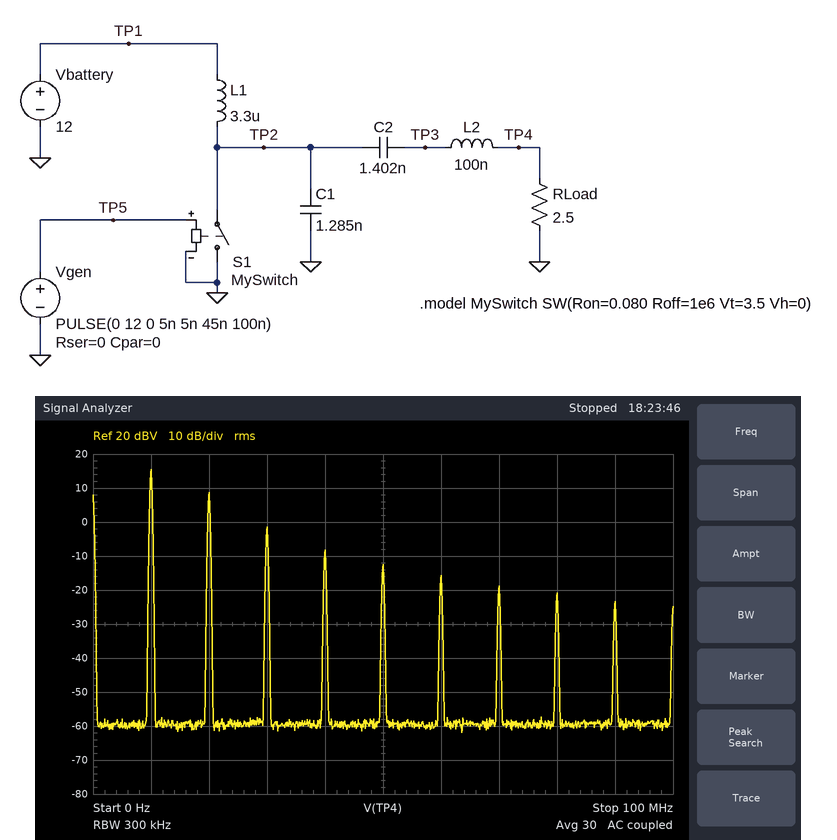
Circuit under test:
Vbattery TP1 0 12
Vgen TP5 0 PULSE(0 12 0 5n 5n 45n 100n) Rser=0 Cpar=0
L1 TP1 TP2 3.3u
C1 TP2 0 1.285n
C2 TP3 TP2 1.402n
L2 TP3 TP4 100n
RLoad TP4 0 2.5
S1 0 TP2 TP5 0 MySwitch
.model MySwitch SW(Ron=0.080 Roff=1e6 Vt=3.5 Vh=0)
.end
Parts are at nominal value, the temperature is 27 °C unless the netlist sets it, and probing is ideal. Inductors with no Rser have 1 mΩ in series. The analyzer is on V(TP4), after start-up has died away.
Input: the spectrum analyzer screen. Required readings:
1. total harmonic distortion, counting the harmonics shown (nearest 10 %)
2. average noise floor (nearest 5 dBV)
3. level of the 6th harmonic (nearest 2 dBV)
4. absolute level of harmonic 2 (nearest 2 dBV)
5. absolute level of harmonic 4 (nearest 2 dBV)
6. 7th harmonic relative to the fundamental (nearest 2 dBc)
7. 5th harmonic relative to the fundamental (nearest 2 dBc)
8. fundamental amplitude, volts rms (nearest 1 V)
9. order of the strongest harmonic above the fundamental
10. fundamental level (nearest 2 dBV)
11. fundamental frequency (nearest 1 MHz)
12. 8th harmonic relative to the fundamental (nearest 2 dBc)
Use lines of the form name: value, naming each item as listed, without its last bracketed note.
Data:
total harmonic distortion, counting the harmonics shown: 50 %
average noise floor: -60 dBV
level of the 6th harmonic: -16 dBV
absolute level of harmonic 2: 8 dBV
absolute level of harmonic 4: -8 dBV
7th harmonic relative to the fundamental: -34 dBc
5th harmonic relative to the fundamental: -28 dBc
fundamental amplitude, volts rms: 6 V
order of the strongest harmonic above the fundamental: 2
fundamental level: 16 dBV
fundamental frequency: 10 MHz
8th harmonic relative to the fundamental: -36 dBc
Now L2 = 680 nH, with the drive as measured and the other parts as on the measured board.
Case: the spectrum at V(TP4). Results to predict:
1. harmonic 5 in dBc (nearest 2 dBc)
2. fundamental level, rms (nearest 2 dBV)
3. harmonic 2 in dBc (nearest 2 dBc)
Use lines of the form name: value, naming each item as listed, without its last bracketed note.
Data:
harmonic 5 in dBc: -34 dBc
fundamental level, rms: 0 dBV
harmonic 2 in dBc: -16 dBc
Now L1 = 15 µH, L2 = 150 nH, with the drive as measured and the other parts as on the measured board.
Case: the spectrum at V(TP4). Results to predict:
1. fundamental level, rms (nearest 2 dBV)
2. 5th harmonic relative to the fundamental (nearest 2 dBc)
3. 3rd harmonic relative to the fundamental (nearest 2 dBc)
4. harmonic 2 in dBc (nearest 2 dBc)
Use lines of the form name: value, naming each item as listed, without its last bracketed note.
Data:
fundamental level, rms: 18 dBV
5th harmonic relative to the fundamental: -36 dBc
3rd harmonic relative to the fundamental: -24 dBc
harmonic 2 in dBc: -22 dBc
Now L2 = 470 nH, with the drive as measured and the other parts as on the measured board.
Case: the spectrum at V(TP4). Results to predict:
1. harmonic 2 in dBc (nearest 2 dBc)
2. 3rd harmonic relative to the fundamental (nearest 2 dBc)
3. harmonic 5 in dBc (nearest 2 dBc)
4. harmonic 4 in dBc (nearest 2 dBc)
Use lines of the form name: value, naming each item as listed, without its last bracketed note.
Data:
harmonic 2 in dBc: -18 dBc
3rd harmonic relative to the fundamental: -28 dBc
harmonic 5 in dBc: -38 dBc
harmonic 4 in dBc: -32 dBc
